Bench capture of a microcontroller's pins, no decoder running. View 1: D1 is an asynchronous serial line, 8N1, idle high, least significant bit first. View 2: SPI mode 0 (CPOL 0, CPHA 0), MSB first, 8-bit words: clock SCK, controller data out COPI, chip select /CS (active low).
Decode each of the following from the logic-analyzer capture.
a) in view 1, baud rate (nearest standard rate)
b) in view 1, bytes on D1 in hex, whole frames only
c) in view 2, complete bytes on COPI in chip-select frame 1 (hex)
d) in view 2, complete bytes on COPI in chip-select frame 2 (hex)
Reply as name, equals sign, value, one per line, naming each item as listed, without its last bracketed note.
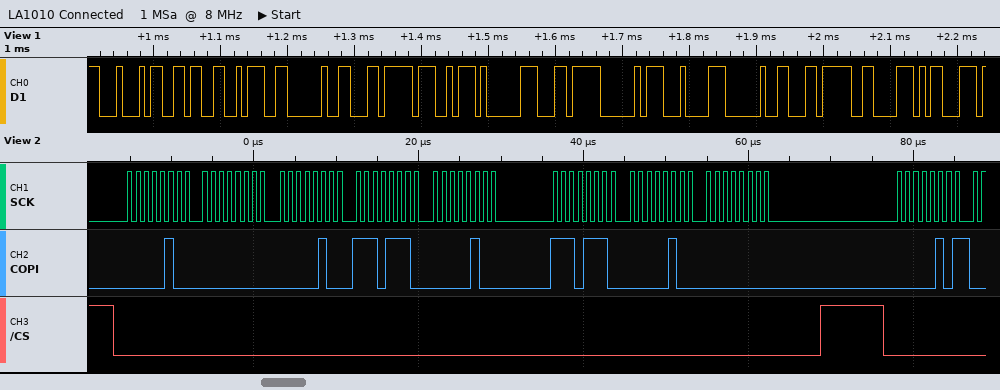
in view 1, baud rate = 115200 baud
in view 1, bytes on D1 in hex, whole frames only = 44 36 3A 20 EC A7 81 EC A0 84 20 EC 86 8D
in view 2, complete bytes on COPI in chip-select frame 1 = 0x04 0x00 0x04 0xEE 0x04 0xEE 0x04 0x00
in view 2, complete bytes on COPI in chip-select frame 2 = 0x05
